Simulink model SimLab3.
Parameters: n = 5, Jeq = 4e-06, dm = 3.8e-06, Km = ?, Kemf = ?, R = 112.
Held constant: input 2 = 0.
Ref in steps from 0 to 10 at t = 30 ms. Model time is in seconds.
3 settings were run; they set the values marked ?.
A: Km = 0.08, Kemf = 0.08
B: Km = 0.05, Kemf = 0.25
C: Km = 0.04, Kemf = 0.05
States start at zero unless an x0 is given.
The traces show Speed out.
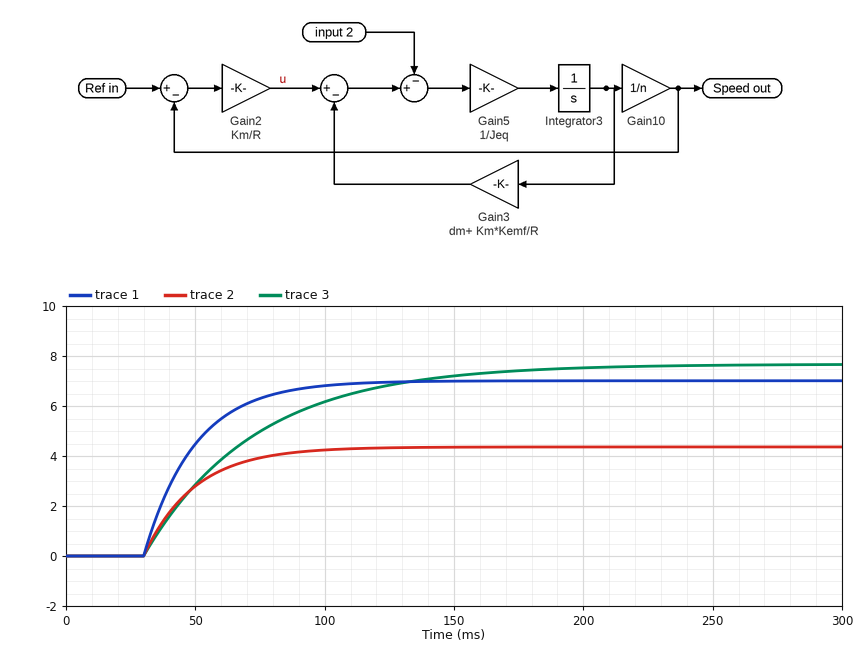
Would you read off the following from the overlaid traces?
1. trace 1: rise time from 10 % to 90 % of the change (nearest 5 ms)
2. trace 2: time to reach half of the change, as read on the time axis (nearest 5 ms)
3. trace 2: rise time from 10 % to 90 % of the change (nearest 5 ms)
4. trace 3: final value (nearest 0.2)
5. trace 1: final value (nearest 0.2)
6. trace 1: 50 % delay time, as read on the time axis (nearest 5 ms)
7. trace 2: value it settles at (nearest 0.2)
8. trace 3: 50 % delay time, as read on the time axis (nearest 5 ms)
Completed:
45 ms
45 ms
45 ms
7.6
7.0
45 ms
4.4
60 ms
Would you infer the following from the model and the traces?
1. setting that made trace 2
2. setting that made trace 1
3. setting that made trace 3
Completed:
B
A
C
